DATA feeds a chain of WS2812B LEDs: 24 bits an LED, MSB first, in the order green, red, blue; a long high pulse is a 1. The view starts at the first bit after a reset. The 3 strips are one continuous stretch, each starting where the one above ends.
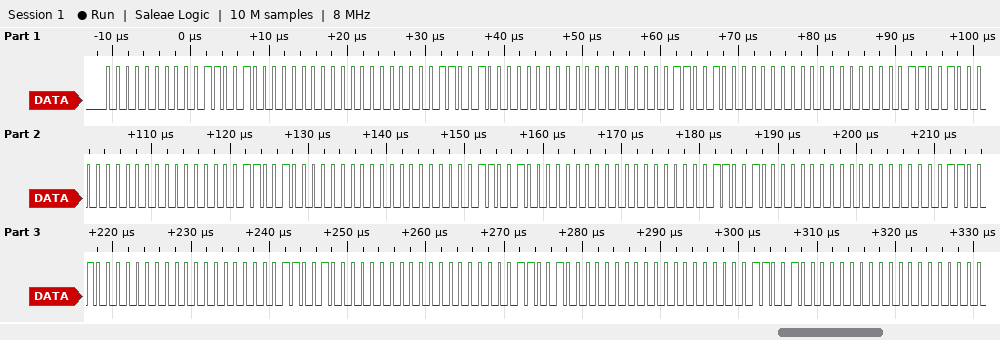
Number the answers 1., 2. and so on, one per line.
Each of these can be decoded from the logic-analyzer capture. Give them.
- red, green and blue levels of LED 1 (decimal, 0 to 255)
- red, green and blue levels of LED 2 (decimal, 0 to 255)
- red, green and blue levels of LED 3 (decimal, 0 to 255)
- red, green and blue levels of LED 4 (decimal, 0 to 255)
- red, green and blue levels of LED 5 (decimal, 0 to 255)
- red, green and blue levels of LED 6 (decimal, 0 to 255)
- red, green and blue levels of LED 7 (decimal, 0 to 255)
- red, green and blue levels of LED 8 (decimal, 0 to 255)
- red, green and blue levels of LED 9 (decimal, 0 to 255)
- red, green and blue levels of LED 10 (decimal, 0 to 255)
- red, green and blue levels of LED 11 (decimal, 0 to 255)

1. 50, 0, 0
2. 50, 0, 0
3. 50, 0, 0
4. 50, 0, 0
5. 50, 0, 0
6. 50, 0, 0
7. 50, 0, 0
8. 50, 0, 0
9. 50, 0, 0
10. 50, 0, 0
11. 50, 0, 0
